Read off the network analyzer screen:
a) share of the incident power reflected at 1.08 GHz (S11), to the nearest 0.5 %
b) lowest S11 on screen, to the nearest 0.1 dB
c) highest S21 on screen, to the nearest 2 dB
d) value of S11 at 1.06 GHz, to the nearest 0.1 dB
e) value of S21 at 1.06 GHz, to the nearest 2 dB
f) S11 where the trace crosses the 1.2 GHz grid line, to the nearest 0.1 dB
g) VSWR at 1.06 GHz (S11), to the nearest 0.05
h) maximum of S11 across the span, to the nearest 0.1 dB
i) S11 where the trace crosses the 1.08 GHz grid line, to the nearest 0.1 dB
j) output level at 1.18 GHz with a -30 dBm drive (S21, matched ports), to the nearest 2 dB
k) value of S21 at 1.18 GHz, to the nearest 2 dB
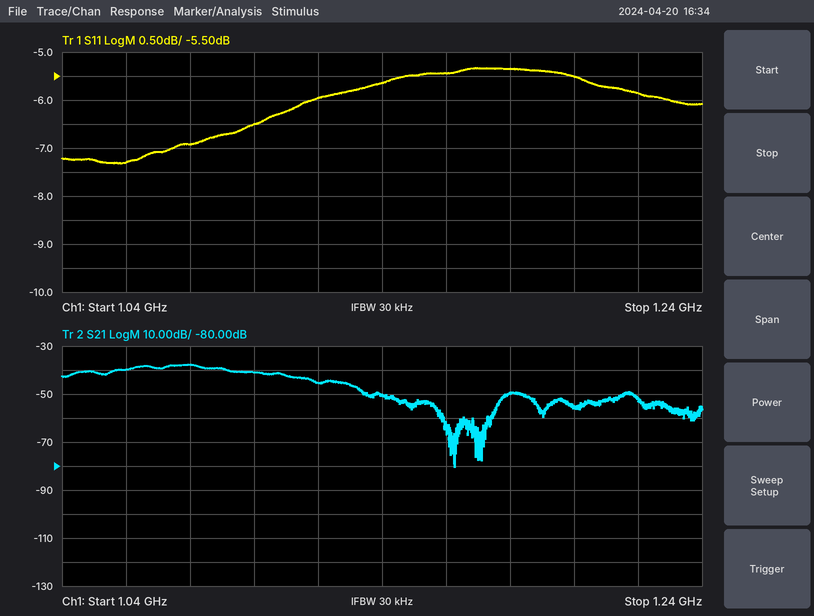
20.5 %
-7.3 dB
-38 dB
-7.3 dB
-40 dB
-5.5 dB
2.50
-5.3 dB
-6.9 dB
-80 dBm
-50 dB
